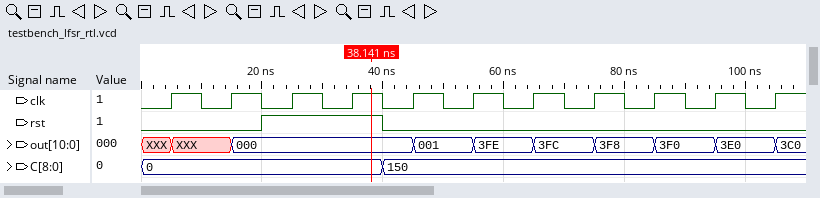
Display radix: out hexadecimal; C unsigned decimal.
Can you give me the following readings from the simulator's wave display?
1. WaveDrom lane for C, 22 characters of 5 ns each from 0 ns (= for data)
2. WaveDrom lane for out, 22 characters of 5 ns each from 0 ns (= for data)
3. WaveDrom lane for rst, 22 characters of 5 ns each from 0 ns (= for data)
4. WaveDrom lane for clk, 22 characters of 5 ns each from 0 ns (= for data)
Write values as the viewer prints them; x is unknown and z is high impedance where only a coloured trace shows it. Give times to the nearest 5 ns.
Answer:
{name: 'C', wave: '=.......=.............', data: '0 150'}
{name: 'out', wave: 'x=.=.....=.=.=.=.=.=.=', data: 'XXX 000 001 3FE 3FC 3F8 3F0 3E0 3C0'}
{name: 'rst', wave: '0...1...0.............'}
{name: 'clk', wave: '0101010101010101010101'}
